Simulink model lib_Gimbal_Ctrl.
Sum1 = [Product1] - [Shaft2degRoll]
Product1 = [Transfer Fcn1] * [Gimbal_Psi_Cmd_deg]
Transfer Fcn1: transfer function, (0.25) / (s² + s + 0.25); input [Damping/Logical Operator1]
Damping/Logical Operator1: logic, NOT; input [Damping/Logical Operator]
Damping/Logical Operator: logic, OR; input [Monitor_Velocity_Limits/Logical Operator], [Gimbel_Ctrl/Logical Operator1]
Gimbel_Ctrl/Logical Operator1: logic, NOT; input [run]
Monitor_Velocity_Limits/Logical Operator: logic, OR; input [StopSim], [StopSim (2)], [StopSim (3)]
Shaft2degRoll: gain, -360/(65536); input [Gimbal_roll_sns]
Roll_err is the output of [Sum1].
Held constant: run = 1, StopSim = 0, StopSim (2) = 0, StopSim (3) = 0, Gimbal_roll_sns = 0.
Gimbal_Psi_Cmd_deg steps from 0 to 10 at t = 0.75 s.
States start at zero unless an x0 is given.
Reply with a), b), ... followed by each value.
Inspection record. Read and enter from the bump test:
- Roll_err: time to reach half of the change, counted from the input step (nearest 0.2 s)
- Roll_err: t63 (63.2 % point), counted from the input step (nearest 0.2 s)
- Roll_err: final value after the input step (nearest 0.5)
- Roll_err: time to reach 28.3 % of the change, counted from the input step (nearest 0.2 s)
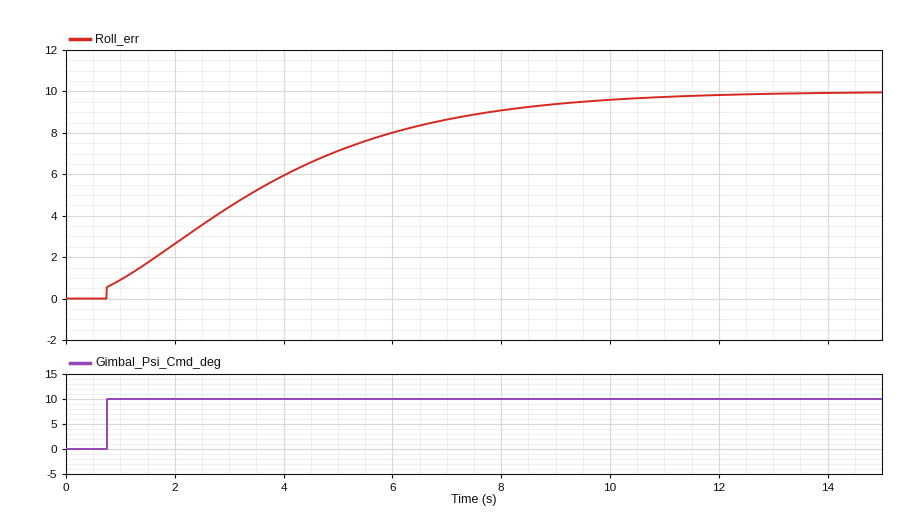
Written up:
a) 2.6 s
b) 3.6 s
c) 10.0
d) 1.4 s
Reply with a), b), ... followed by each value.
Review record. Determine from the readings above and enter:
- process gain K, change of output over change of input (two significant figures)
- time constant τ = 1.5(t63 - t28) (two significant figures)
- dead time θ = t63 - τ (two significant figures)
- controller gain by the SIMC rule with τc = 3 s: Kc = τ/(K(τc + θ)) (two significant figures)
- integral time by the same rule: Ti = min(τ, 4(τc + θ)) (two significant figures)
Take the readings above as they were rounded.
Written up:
a) 1.0
b) 3.3 s
c) 0.30 s
d) 1.0
e) 3.3 s
